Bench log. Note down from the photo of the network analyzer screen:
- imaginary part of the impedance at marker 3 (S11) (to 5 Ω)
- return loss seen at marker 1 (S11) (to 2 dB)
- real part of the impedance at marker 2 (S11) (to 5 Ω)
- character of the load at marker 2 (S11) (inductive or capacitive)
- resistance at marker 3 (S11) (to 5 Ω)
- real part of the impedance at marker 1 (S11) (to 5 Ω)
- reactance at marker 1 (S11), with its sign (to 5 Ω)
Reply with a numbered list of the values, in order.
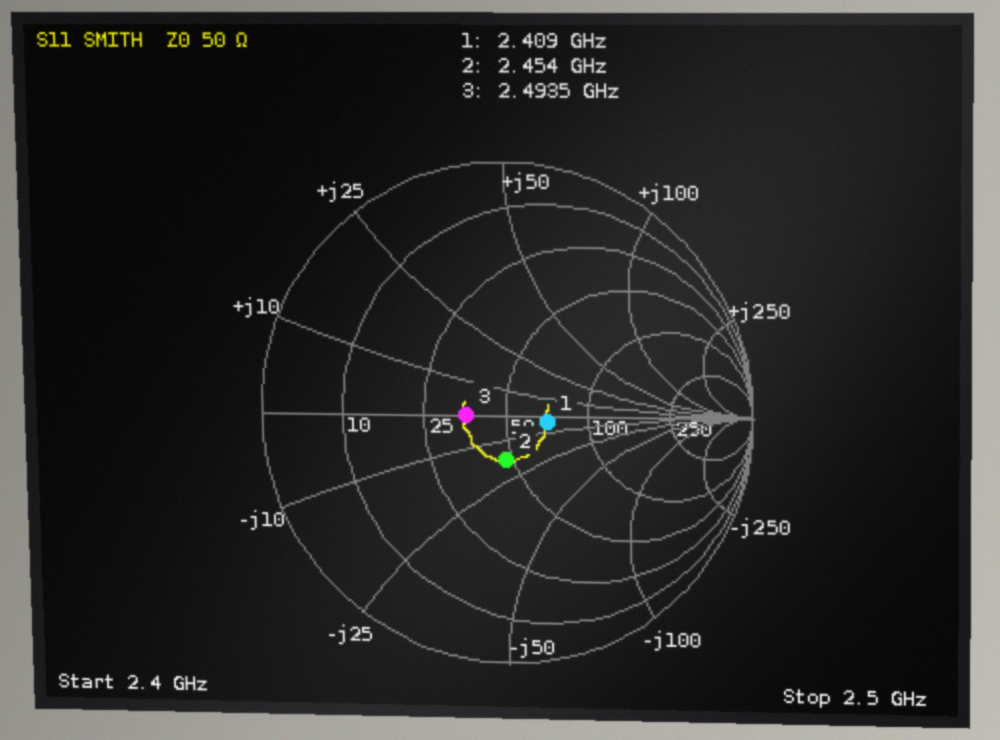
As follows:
1. 0 Ω
2. 16 dB
3. 45 Ω
4. capacitive
5. 35 Ω
6. 70 Ω
7. -5 Ω
